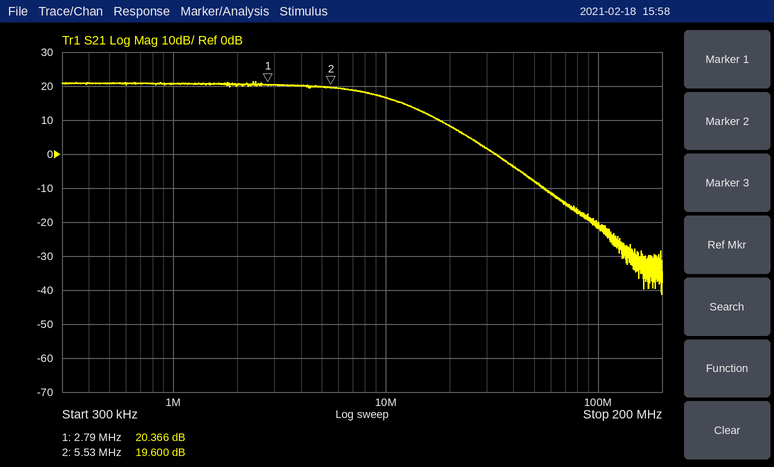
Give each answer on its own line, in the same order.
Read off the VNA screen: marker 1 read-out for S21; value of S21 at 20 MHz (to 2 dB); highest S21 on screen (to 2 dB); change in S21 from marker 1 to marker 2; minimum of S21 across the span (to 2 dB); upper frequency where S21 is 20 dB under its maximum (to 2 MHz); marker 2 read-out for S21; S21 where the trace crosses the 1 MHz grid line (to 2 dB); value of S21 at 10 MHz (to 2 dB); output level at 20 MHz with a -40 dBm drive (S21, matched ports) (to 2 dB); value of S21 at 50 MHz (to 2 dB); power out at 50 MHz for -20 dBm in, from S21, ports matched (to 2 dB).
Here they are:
20.366 dB
8 dB
22 dB
-0.766 dB
-42 dB
30 MHz
19.600 dB
20 dB
16 dB
-32 dBm
-8 dB
-28 dBm
